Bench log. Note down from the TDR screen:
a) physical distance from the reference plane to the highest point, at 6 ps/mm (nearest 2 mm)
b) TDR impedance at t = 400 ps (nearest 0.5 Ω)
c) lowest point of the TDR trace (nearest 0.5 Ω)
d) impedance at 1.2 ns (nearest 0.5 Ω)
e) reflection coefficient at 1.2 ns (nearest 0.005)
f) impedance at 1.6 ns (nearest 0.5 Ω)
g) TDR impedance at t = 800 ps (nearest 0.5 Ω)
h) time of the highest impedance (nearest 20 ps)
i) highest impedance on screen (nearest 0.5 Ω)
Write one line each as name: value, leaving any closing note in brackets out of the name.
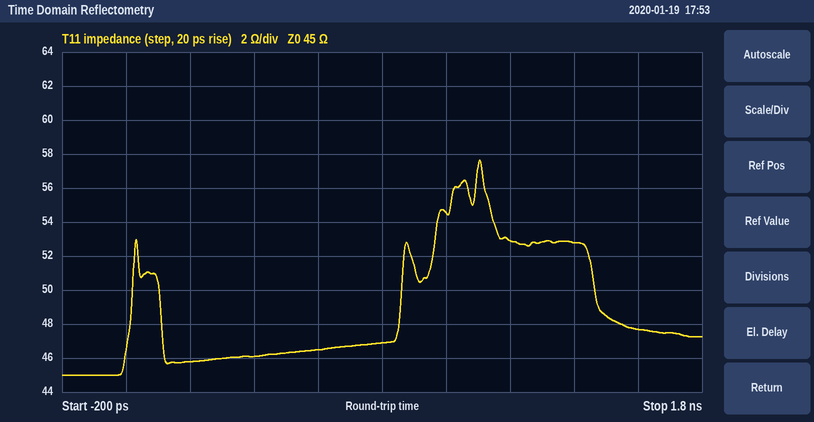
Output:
physical distance from the reference plane to the highest point, at 6 ps/mm: 92 mm
TDR impedance at t = 400 ps: 46.0 Ω
lowest point of the TDR trace: 45.0 Ω
impedance at 1.2 ns: 53.0 Ω
reflection coefficient at 1.2 ns: +0.080
impedance at 1.6 ns: 47.5 Ω
TDR impedance at t = 800 ps: 47.0 Ω
time of the highest impedance: 1.10 ns
highest impedance on screen: 57.5 Ω
